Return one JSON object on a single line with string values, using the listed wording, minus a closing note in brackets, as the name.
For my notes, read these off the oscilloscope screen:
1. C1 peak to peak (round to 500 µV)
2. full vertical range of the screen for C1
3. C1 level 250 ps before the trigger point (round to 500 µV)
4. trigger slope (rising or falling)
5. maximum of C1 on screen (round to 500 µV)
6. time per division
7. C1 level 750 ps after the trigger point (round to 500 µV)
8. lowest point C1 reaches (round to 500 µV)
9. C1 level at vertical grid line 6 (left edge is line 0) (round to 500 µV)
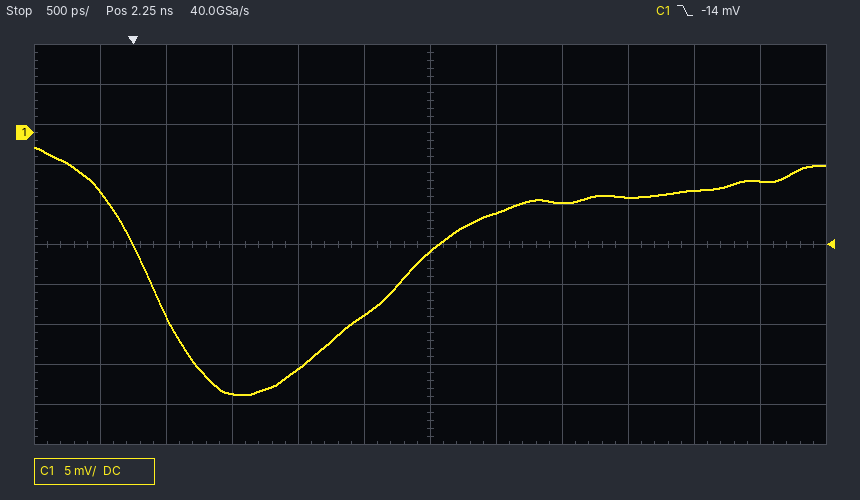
{"C1 peak to peak": "31.0 mV", "full vertical range of the screen for C1": "50 mV", "C1 level 250 ps before the trigger point": "-7.5 mV", "trigger slope": "falling", "maximum of C1 on screen": "-2.0 mV", "time per division": "500 ps", "C1 level 750 ps after the trigger point": "-32.5 mV", "lowest point C1 reaches": "-33.0 mV", "C1 level at vertical grid line 6 (left edge is line 0)": "-15.0 mV"}
